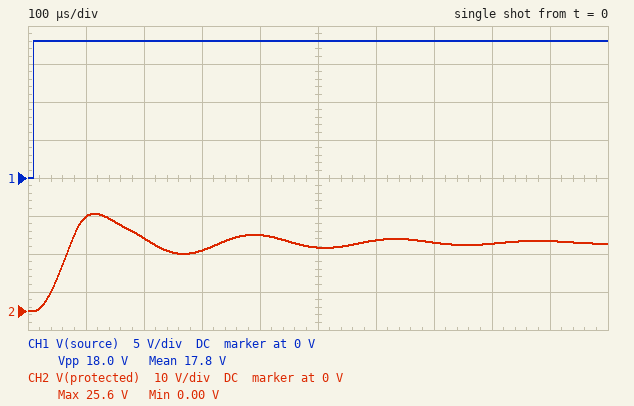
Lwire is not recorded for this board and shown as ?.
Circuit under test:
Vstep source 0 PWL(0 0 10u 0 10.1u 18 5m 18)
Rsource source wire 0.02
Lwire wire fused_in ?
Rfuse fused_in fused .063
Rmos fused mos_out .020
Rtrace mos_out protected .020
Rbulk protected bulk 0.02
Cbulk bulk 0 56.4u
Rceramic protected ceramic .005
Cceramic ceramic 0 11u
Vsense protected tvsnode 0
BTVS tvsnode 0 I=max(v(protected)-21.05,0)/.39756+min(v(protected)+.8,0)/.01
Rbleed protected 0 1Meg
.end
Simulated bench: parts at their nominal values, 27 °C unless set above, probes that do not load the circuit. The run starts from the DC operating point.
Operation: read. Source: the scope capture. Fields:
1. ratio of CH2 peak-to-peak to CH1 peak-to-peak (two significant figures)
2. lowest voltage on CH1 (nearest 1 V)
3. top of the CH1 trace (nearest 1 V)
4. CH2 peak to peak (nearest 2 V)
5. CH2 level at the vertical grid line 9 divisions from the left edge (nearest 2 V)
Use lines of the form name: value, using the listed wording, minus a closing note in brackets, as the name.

ratio of CH2 peak-to-peak to CH1 peak-to-peak: 1.4
lowest voltage on CH1: 0 V
top of the CH1 trace: 18 V
CH2 peak to peak: 26 V
CH2 level at the vertical grid line 9 divisions from the left edge: 18 V
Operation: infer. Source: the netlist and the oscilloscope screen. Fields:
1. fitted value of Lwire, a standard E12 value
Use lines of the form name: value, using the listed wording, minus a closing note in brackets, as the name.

fitted value of Lwire, a standard E12 value: 22 µH
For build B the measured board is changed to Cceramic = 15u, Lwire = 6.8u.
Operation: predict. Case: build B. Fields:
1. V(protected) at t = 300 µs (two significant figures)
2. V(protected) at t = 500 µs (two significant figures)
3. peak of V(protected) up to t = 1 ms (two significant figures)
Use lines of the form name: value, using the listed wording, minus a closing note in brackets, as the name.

V(protected) at t = 300 µs: 17 V
V(protected) at t = 500 µs: 18 V
peak of V(protected) up to t = 1 ms: 25 V
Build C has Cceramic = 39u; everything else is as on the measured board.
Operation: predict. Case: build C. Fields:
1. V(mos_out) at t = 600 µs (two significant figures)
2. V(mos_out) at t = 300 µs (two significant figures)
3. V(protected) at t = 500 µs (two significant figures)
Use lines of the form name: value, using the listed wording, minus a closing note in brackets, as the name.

V(mos_out) at t = 600 µs: 17 V
V(mos_out) at t = 300 µs: 15 V
V(protected) at t = 500 µs: 19 V
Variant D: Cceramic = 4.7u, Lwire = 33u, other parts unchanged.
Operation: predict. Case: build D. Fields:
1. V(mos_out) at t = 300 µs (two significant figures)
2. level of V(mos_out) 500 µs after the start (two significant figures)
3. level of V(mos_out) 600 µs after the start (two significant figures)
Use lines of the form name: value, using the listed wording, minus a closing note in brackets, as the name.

V(mos_out) at t = 300 µs: 15 V
level of V(mos_out) 500 µs after the start: 19 V
level of V(mos_out) 600 µs after the start: 16 V
